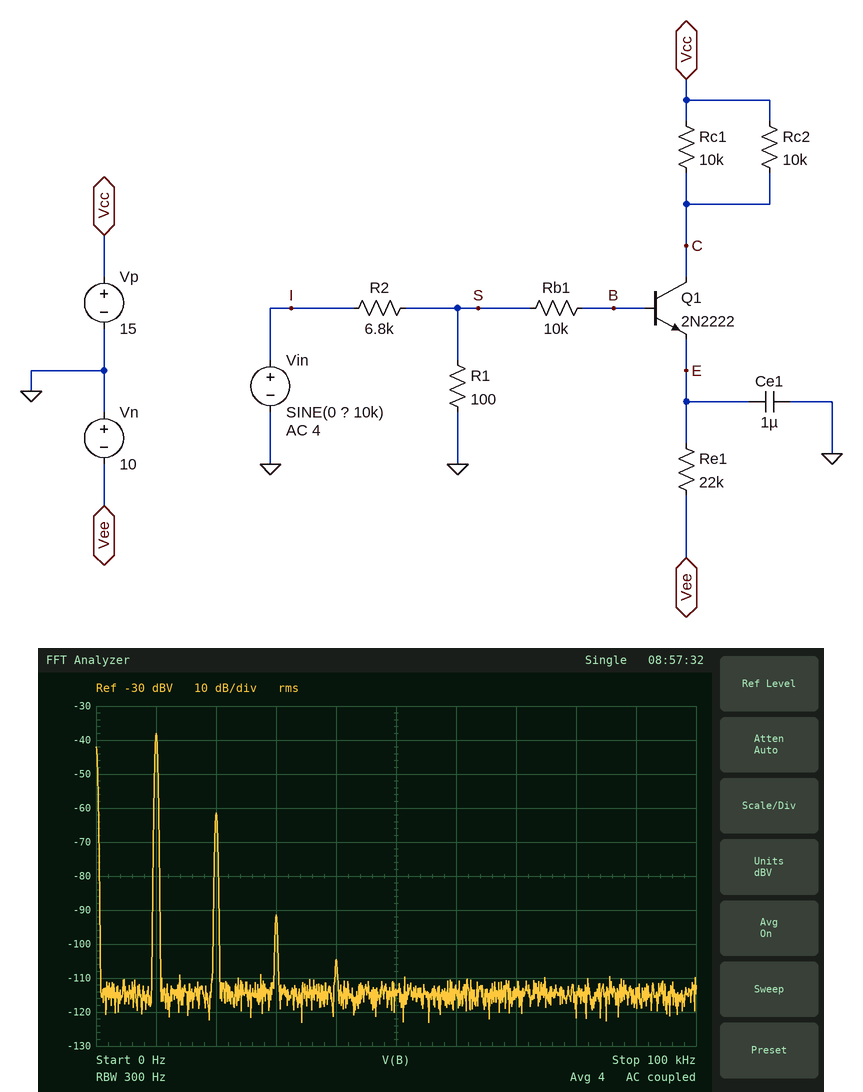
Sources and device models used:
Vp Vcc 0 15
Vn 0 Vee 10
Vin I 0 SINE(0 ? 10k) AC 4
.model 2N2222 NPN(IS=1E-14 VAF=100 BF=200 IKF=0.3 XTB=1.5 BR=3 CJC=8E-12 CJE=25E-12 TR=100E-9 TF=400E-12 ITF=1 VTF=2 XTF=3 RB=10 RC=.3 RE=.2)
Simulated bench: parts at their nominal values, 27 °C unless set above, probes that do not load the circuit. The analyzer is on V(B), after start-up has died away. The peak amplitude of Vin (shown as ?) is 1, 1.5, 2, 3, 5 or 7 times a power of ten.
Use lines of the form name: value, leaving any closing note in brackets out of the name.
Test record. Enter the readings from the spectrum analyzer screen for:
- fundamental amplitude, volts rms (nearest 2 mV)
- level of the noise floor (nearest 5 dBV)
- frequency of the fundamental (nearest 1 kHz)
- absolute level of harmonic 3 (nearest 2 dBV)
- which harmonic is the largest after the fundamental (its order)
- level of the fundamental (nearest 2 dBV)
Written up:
fundamental amplitude, volts rms: 12 mV
level of the noise floor: -115 dBV
frequency of the fundamental: 10 kHz
absolute level of harmonic 3: -92 dBV
which harmonic is the largest after the fundamental: 2
level of the fundamental: -38 dBV
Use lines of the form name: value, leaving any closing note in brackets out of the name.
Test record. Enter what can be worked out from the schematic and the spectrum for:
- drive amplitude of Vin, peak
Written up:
drive amplitude of Vin, peak: 2 V
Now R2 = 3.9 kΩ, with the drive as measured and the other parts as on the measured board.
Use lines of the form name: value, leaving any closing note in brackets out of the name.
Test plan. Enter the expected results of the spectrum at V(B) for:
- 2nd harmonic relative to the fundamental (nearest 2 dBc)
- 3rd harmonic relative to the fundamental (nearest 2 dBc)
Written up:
2nd harmonic relative to the fundamental: -20 dBc
3rd harmonic relative to the fundamental: -48 dBc
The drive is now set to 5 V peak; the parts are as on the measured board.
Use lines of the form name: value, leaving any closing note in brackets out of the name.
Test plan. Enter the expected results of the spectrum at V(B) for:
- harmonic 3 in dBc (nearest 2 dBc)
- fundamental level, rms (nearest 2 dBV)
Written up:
harmonic 3 in dBc: -46 dBc
fundamental level, rms: -30 dBV
